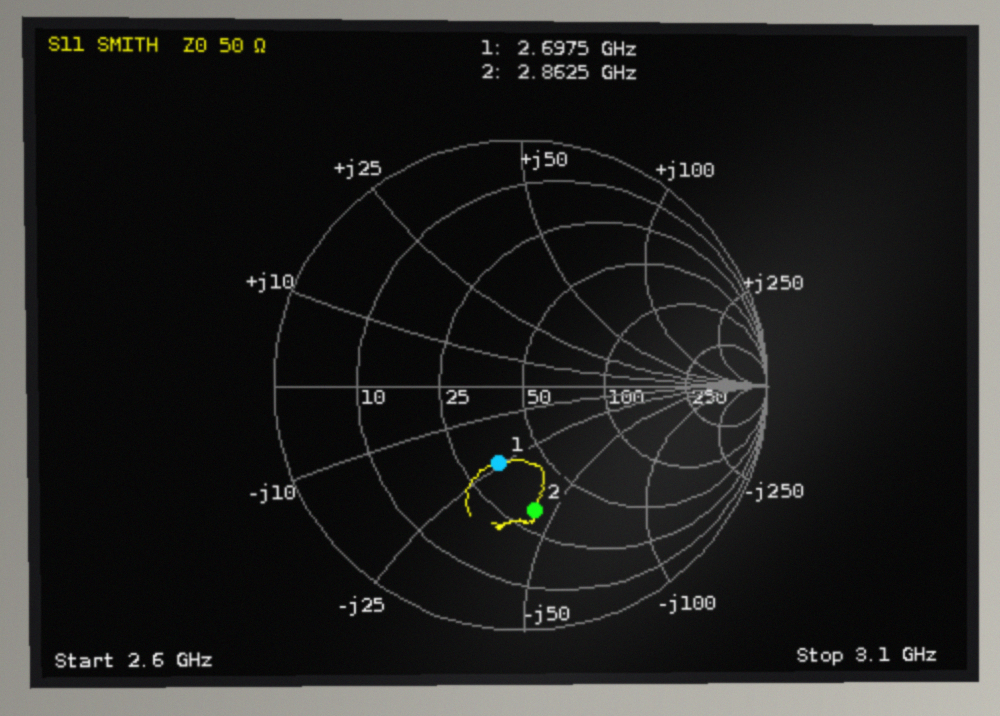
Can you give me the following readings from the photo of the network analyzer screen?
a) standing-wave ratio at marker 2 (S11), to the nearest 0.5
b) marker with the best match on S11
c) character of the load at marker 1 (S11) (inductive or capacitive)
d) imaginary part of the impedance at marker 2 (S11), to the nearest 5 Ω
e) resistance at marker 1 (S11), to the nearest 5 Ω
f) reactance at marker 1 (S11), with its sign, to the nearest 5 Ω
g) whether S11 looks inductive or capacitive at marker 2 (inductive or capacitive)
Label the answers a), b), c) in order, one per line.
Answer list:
a) 3.0
b) marker 1
c) capacitive
d) -45 Ω
e) 35 Ω
f) -25 Ω
g) capacitive
